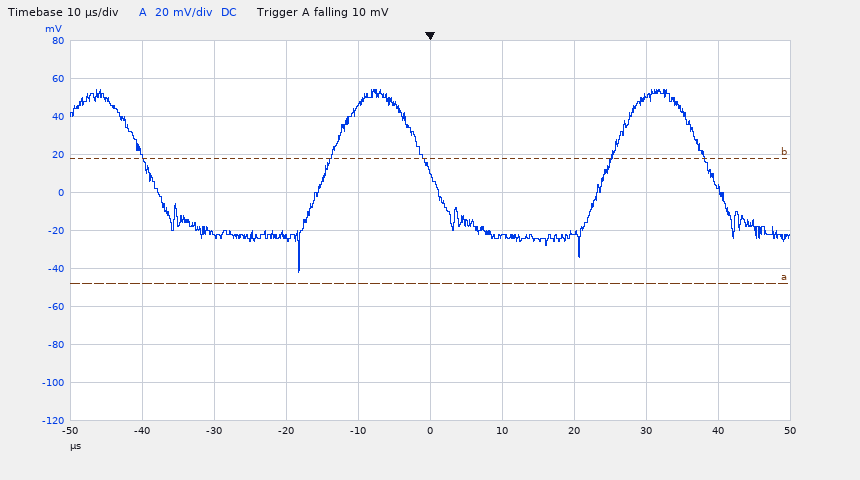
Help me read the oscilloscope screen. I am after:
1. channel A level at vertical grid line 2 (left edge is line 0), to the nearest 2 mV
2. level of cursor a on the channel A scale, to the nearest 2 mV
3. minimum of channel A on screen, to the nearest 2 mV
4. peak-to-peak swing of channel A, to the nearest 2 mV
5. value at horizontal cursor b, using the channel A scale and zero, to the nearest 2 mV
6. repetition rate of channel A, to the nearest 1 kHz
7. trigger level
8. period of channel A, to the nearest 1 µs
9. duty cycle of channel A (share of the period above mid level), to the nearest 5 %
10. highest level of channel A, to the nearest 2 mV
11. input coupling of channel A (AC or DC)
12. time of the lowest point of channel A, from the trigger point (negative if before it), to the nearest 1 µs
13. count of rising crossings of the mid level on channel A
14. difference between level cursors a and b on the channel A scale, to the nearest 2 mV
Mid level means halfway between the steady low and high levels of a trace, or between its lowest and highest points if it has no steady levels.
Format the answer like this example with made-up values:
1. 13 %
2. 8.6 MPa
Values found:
1. -22 mV
2. -48 mV
3. -42 mV
4. 96 mV
5. 18 mV
6. 26 kHz
7. 10 mV
8. 39 µs
9. 40 %
10. 54 mV
11. DC
12. -18 µs
13. 2
14. 66 mV
